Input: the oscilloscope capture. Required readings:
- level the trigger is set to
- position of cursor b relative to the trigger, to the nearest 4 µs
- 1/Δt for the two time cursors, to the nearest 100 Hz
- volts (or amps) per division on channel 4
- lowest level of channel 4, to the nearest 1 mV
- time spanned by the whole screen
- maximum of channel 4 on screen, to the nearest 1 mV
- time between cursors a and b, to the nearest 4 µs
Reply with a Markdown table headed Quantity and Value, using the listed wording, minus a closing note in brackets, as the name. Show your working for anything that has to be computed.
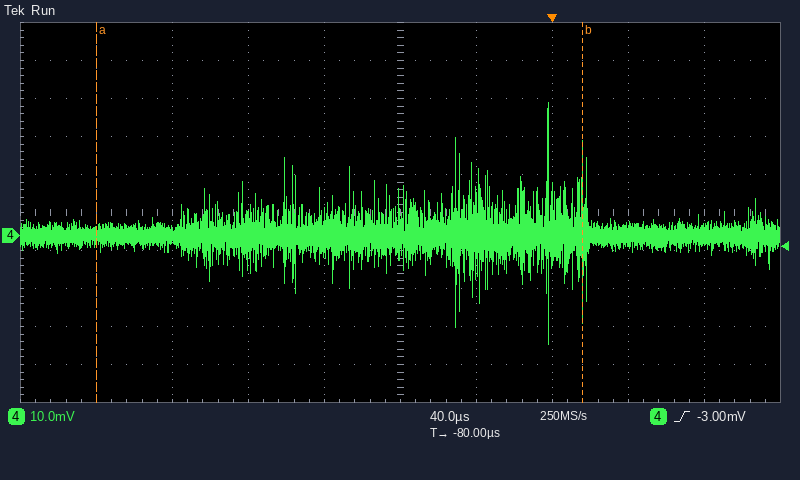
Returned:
| Quantity | Value |
|---|---|
| level the trigger is set to | -3.00 mV |
| position of cursor b relative to the trigger, to the nearest 4 µs | +16 µs |
| 1/Δt for the two time cursors, to the nearest 100 Hz | 1 / 256 µs ≈ 3.9 kHz |
| volts (or amps) per division on channel 4 | 10 mV |
| lowest level of channel 4, to the nearest 1 mV | -29 mV |
| time spanned by the whole screen | 400 µs |
| maximum of channel 4 on screen, to the nearest 1 mV | 35 mV |
| time between cursors a and b, to the nearest 4 µs | 256 µs |
